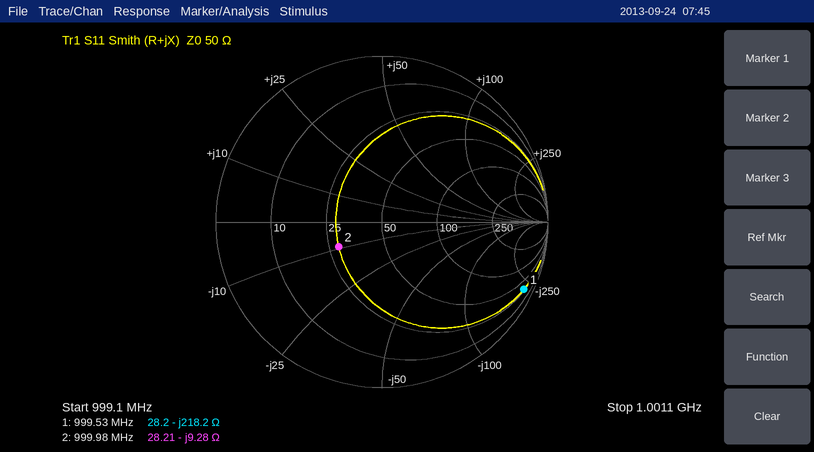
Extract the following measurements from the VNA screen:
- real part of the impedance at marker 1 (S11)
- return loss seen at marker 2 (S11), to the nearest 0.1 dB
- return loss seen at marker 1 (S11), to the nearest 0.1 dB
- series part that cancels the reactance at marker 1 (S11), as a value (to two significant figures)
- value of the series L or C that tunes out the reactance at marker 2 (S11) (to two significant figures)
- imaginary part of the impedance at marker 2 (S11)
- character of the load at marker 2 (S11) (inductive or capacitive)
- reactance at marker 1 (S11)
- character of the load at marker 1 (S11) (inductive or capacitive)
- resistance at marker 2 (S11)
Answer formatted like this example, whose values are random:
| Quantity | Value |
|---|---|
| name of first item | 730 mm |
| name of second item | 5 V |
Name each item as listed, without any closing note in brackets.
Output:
| Quantity | Value |
|---|---|
| real part of the impedance at marker 1 | 28.2 Ω |
| return loss seen at marker 2 (S11), to the nearest 0.1 dB | 10.4 dB |
| return loss seen at marker 1 (S11), to the nearest 0.1 dB | 0.5 dB |
| series part that cancels the reactance at marker 1 (S11), as a value | 35 nH |
| value of the series L or C that tunes out the reactance at marker 2 (S11) | 1.5 nH |
| imaginary part of the impedance at marker 2 | -9.28 Ω |
| character of the load at marker 2 (S11) | capacitive |
| reactance at marker 1 | -218.2 Ω |
| character of the load at marker 1 (S11) | capacitive |
| resistance at marker 2 | 28.21 Ω |
